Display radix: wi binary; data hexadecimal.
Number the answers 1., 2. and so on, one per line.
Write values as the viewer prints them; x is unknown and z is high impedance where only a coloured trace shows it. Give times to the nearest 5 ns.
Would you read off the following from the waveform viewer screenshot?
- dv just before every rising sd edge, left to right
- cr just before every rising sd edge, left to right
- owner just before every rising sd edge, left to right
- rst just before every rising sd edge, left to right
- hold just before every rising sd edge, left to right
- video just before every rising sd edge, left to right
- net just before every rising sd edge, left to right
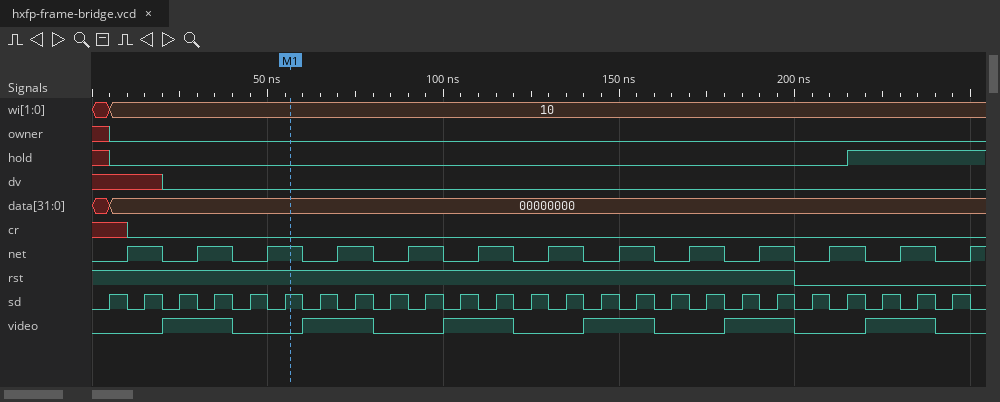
1. x x 0 0 0 0 0 0 0 0 0 0 0 0 0 0 0 0 0 0 0 0 0 0 0
2. x 0 0 0 0 0 0 0 0 0 0 0 0 0 0 0 0 0 0 0 0 0 0 0 0
3. x 0 0 0 0 0 0 0 0 0 0 0 0 0 0 0 0 0 0 0 0 0 0 0 0
4. 1 1 1 1 1 1 1 1 1 1 1 1 1 1 1 1 1 1 1 1 0 0 0 0 0
5. x 0 0 0 0 0 0 0 0 0 0 0 0 0 0 0 0 0 0 0 0 0 1 1 1
6. 0 0 1 1 0 0 1 1 0 0 1 1 0 0 1 1 0 0 1 1 0 0 1 1 0
7. 0 1 0 1 0 1 0 1 0 1 0 1 0 1 0 1 0 1 0 1 0 1 0 1 0
